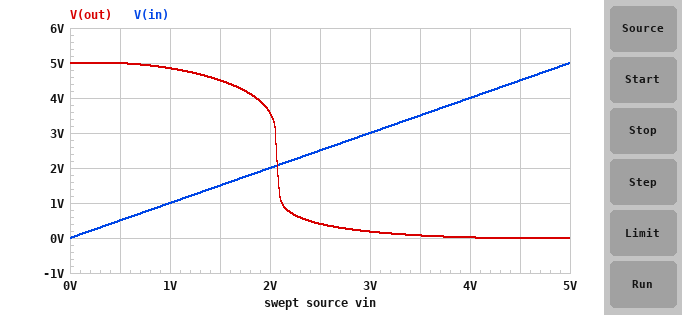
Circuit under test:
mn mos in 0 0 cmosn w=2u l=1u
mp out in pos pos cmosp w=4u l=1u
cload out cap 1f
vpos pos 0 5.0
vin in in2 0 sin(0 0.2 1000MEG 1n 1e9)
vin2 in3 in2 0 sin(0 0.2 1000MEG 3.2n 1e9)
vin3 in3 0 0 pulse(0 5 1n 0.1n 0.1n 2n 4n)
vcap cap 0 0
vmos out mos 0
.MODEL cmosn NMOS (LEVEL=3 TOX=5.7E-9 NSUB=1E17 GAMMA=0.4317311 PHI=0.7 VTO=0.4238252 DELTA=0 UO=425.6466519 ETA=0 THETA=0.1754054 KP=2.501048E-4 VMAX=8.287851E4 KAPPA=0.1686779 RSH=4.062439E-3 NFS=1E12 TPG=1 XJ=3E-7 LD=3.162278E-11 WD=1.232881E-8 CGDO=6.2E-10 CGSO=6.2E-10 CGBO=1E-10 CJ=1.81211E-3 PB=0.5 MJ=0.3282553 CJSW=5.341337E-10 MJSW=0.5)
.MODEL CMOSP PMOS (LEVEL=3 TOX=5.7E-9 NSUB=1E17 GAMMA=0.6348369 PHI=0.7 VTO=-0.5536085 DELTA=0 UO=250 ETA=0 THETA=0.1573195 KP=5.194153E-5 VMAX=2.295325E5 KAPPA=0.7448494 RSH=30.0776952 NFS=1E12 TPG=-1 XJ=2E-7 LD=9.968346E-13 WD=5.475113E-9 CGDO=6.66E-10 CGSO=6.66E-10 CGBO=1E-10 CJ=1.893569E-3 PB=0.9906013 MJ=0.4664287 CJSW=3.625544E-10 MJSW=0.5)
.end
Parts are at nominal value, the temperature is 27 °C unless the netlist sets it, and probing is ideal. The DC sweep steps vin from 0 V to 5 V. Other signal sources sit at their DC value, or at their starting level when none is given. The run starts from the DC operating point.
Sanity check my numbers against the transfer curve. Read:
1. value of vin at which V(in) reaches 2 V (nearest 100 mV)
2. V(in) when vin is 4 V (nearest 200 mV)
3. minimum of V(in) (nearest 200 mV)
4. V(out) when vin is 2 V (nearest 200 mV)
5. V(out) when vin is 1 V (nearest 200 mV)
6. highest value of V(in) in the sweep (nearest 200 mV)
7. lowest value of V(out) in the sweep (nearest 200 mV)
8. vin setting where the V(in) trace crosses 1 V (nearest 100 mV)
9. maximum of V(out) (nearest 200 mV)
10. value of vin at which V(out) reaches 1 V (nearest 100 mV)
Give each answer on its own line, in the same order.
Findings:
2.0 V
4.0 V
0 V
3.6 V
4.8 V
5.0 V
0 V
1.0 V
5.0 V
2.1 V
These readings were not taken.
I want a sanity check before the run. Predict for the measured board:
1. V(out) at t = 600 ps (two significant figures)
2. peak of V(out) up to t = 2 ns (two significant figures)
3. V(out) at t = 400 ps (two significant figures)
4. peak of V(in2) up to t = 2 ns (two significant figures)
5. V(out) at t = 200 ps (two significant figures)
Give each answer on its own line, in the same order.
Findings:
5.0 V
5.6 V
5.0 V
5.0 V
5.0 V
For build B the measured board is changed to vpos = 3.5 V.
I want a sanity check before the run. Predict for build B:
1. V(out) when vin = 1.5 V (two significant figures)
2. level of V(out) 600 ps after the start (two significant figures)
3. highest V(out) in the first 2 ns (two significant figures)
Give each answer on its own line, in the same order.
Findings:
520 mV
3.5 V
4.1 V
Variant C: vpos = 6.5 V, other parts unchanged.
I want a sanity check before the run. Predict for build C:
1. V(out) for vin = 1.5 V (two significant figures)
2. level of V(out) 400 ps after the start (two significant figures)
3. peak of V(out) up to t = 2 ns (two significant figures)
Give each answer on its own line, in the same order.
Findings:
6.1 V
6.5 V
7.1 V
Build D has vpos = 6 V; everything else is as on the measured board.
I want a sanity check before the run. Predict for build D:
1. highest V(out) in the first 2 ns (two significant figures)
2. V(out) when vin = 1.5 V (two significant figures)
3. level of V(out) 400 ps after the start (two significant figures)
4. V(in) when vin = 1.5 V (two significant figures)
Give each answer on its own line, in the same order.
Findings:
6.6 V
5.6 V
6.0 V
1.5 V
